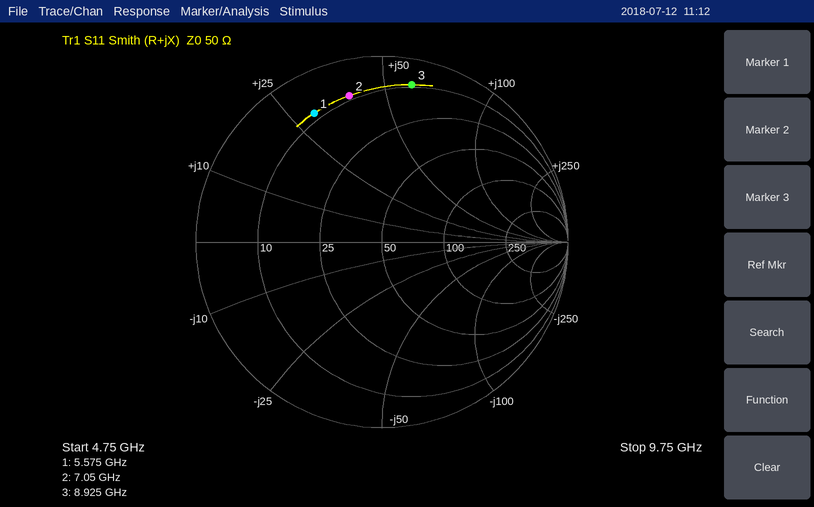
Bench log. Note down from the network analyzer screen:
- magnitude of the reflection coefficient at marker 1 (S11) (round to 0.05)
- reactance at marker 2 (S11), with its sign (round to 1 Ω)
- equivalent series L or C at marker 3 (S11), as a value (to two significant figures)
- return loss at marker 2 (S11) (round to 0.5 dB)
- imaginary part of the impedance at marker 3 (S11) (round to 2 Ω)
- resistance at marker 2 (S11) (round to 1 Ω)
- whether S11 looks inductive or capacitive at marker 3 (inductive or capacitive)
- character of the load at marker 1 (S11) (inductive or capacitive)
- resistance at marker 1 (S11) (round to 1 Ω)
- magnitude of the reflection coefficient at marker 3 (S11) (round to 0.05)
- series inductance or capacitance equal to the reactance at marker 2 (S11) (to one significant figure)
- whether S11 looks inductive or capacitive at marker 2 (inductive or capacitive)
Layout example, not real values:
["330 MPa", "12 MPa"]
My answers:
["0.80", "+39 Ω", "1.1 nH", "2.0 dB", "+60 Ω", "9 Ω", "inductive", "inductive", "8 Ω", "0.85", "900 pH", "inductive"]
